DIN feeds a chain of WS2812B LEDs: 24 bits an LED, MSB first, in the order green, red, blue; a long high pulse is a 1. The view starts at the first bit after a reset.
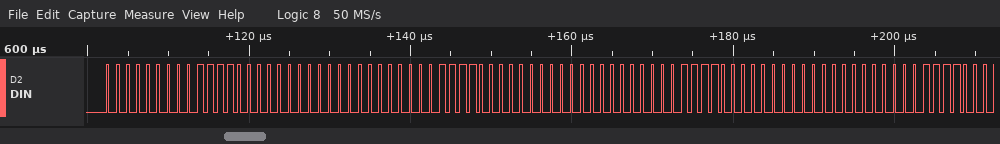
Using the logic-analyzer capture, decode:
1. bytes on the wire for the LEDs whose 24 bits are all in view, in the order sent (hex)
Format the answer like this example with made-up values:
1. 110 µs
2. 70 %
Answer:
1. 00 78 00 00 78 00 00 78 00
